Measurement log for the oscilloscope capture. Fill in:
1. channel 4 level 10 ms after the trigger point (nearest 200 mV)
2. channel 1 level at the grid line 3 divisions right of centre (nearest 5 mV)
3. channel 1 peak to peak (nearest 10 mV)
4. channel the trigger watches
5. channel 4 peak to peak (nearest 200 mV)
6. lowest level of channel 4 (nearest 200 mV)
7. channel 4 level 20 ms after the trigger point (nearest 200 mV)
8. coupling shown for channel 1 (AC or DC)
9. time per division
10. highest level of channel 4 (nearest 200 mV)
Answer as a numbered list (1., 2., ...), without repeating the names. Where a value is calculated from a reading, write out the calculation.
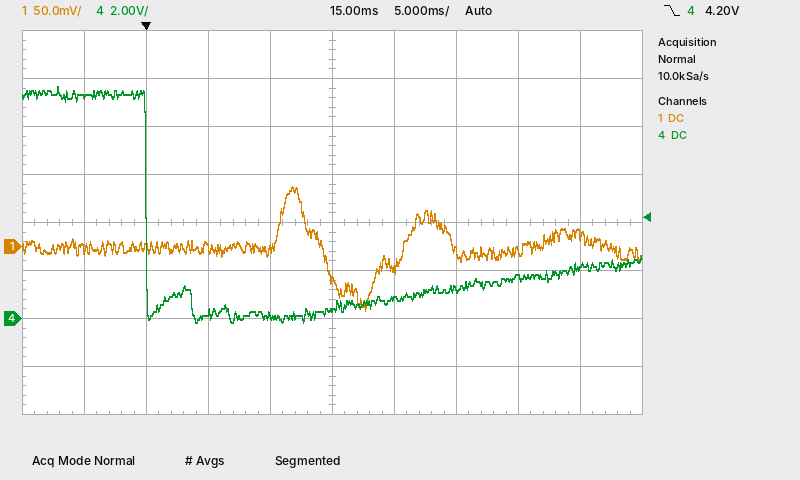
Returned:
1. 200 mV
2. -5 mV
3. 130 mV
4. channel 4
5. 9.6 V − (-200 mV) = 9.8 V
6. -200 mV
7. 800 mV
8. DC
9. 5 ms
10. 9.6 V
